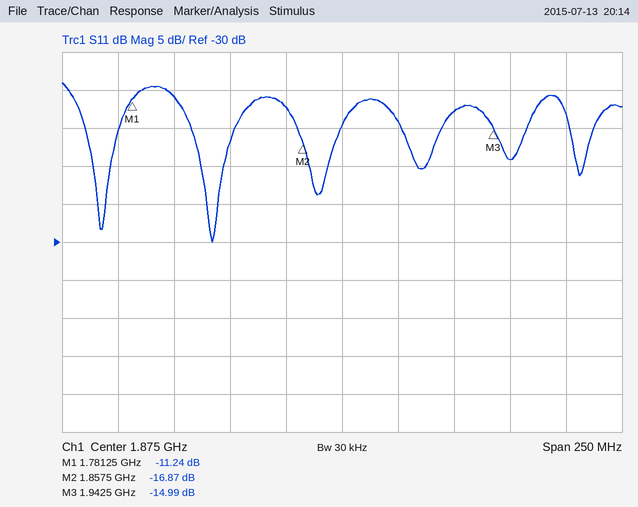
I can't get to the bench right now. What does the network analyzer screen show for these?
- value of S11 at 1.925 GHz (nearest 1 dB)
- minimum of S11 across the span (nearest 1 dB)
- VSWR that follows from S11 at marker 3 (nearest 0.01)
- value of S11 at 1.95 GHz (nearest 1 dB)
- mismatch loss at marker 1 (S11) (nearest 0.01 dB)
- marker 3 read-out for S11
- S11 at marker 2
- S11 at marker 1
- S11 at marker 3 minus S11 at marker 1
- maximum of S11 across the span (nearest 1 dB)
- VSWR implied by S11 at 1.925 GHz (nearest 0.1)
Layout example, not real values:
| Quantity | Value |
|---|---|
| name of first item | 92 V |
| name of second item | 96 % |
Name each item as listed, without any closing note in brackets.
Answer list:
| Quantity | Value |
|---|---|
| value of S11 at 1.925 GHz | -13 dB |
| minimum of S11 across the span | -30 dB |
| VSWR that follows from S11 at marker 3 | 1.43 |
| value of S11 at 1.95 GHz | -19 dB |
| mismatch loss at marker 1 (S11) | 0.34 dB |
| marker 3 read-out for S11 | -14.99 dB |
| S11 at marker 2 | -16.87 dB |
| S11 at marker 1 | -11.24 dB |
| S11 at marker 3 minus S11 at marker 1 | -3.75 dB |
| maximum of S11 across the span | -9 dB |
| VSWR implied by S11 at 1.925 GHz | 1.6 |
